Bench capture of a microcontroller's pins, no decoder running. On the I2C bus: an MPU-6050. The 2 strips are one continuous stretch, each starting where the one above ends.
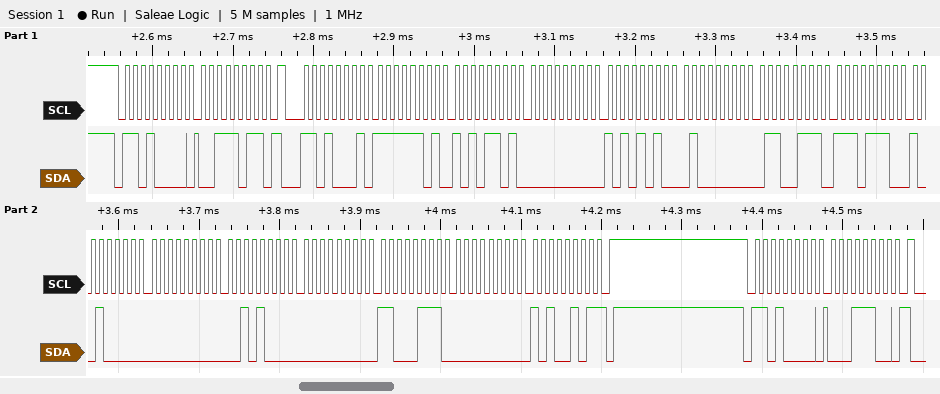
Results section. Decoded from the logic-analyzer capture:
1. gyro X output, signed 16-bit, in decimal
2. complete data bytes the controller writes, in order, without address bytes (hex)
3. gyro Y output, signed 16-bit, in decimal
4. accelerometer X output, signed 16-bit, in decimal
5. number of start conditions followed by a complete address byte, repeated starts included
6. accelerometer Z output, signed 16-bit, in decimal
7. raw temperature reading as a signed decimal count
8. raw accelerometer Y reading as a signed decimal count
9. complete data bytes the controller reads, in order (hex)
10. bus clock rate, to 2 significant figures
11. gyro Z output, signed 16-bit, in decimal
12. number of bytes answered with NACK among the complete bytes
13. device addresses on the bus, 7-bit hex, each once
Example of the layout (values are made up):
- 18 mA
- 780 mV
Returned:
- 40
- 3B 1C
- 199
- -595
- 3
- 16487
- -4464
- 170
- FD AD 00 AA 40 67 EE 90 00 28 00 C7 00 A5
- 100 kHz
- 165
- 1
- 0x68
